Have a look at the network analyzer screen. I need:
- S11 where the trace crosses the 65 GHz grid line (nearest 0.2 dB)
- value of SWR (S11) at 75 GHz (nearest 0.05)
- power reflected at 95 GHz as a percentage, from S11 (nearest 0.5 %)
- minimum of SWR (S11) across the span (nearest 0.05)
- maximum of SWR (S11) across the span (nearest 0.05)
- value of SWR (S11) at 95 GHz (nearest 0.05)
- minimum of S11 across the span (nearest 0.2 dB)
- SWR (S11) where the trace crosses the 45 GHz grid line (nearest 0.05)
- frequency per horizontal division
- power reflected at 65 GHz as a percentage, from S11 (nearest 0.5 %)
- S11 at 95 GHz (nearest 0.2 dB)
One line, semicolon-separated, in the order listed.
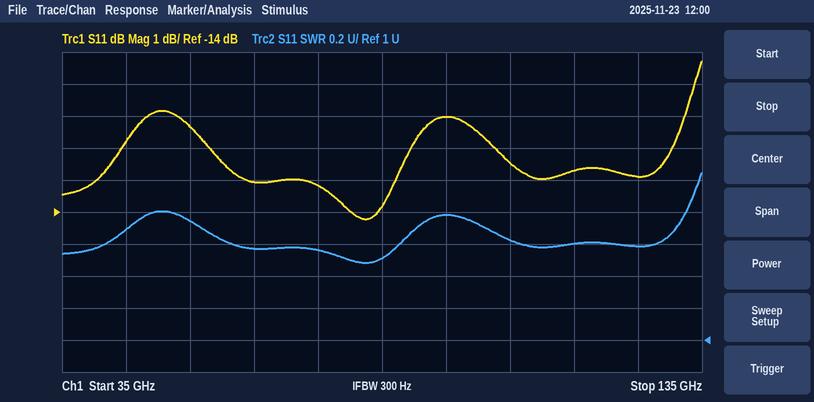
-13.0 dB; 1.55; 8.0 %; 1.50; 2.05; 1.80; -14.2 dB; 1.70; 10 GHz; 5.0 %; -11.0 dB
